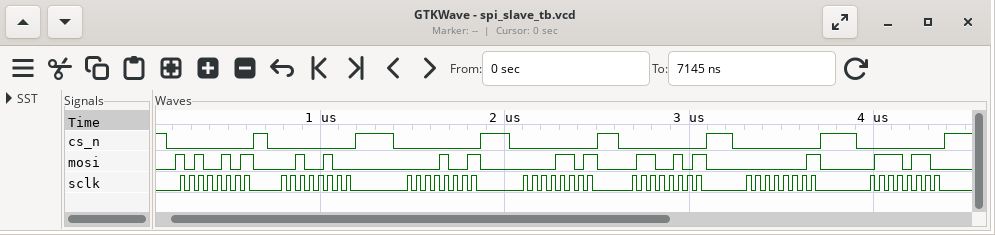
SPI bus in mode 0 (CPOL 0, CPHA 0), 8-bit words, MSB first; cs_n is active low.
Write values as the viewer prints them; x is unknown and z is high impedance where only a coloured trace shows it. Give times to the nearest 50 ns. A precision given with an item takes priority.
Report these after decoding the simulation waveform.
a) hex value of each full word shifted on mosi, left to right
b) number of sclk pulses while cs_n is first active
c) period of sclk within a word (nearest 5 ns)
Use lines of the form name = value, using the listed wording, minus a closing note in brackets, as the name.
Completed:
hex value of each full word shifted on mosi, left to right = A5, 24, 09, 0D, 65, 01, 76
number of sclk pulses while cs_n is first active = 8
period of sclk within a word = 50 ns
